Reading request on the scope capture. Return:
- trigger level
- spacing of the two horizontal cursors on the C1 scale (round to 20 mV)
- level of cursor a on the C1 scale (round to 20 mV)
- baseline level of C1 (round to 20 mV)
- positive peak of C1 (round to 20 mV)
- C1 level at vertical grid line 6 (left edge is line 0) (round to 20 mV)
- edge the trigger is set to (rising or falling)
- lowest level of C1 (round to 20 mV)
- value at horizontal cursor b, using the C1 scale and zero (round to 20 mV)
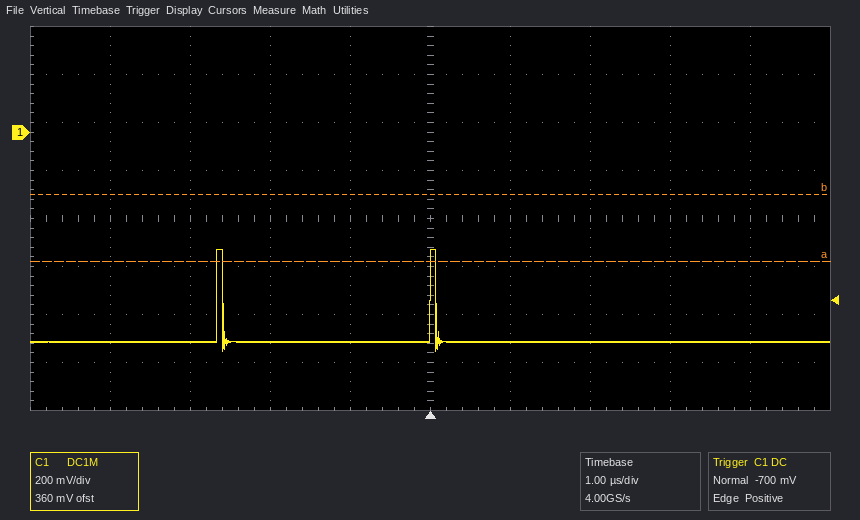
-700 mV
280 mV
-540 mV
-880 mV
-480 mV
-880 mV
rising
-920 mV
-260 mV
